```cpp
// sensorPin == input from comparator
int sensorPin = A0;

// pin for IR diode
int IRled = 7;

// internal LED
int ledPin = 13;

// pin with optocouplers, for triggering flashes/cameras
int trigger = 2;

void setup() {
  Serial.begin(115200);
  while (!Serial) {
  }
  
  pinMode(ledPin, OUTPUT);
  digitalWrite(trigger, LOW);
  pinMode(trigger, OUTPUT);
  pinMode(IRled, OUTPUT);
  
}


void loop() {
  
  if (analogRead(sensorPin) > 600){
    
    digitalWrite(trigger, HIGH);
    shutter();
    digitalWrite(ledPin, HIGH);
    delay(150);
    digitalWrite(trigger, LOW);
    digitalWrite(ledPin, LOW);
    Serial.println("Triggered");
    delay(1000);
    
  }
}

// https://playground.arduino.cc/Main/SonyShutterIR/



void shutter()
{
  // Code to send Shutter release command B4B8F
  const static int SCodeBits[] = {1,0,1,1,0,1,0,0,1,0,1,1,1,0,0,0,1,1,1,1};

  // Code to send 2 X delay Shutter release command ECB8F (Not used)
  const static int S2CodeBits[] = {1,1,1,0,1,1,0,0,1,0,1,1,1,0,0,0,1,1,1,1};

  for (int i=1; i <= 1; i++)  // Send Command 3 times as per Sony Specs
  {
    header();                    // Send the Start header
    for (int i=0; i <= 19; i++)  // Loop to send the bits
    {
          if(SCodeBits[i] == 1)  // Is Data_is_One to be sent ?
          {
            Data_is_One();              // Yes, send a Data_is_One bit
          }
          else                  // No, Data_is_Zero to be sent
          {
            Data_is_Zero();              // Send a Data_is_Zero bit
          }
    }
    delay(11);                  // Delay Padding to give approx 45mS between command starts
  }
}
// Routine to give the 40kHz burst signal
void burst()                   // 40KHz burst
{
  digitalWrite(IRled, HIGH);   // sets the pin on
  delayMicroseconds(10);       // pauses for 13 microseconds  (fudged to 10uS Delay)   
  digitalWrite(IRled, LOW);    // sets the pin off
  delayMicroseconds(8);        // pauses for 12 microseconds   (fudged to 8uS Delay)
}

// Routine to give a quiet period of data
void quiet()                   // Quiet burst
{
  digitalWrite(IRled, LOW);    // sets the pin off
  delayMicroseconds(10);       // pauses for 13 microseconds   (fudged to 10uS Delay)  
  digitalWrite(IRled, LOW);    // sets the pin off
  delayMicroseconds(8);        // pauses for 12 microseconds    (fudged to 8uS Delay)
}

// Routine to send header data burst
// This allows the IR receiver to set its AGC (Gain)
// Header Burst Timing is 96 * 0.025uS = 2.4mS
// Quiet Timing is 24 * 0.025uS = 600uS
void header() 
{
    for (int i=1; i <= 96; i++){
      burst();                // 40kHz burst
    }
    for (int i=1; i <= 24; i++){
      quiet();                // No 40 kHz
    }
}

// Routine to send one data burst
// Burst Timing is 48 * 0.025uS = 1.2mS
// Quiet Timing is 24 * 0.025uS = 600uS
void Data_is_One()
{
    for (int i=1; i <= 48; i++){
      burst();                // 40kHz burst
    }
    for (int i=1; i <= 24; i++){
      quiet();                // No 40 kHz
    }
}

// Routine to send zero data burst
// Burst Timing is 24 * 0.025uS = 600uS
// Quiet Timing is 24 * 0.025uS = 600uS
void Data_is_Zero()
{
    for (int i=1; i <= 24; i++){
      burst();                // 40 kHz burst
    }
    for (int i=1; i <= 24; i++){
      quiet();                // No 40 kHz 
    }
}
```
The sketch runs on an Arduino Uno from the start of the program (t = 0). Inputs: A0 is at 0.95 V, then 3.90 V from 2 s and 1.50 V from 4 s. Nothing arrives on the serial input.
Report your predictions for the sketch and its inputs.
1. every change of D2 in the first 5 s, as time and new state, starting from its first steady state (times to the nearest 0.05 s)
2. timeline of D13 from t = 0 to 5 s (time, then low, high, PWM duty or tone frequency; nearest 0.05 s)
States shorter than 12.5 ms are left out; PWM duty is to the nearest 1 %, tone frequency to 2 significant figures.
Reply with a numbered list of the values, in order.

1. 0 s low; 2 s high; 2.2 s low; 3.2 s high; 3.4 s low
2. 0 s low; 2.05 s high; 2.2 s low; 3.25 s high; 3.4 s low
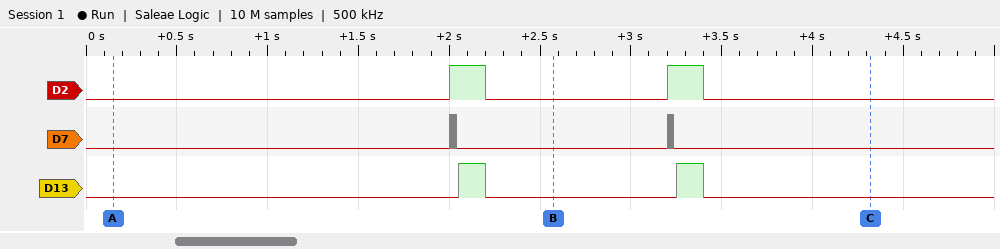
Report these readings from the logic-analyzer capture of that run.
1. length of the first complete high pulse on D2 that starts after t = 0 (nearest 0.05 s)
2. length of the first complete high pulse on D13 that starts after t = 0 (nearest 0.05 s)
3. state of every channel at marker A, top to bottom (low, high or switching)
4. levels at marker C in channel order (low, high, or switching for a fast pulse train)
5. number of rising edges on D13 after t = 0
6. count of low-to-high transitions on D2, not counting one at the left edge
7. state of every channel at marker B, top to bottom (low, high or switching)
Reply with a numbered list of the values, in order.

1. 0.20 s
2. 0.15 s
3. D2 low, D7 low, D13 low
4. D2 low, D7 low, D13 low
5. 2
6. 2
7. D2 low, D7 low, D13 low
